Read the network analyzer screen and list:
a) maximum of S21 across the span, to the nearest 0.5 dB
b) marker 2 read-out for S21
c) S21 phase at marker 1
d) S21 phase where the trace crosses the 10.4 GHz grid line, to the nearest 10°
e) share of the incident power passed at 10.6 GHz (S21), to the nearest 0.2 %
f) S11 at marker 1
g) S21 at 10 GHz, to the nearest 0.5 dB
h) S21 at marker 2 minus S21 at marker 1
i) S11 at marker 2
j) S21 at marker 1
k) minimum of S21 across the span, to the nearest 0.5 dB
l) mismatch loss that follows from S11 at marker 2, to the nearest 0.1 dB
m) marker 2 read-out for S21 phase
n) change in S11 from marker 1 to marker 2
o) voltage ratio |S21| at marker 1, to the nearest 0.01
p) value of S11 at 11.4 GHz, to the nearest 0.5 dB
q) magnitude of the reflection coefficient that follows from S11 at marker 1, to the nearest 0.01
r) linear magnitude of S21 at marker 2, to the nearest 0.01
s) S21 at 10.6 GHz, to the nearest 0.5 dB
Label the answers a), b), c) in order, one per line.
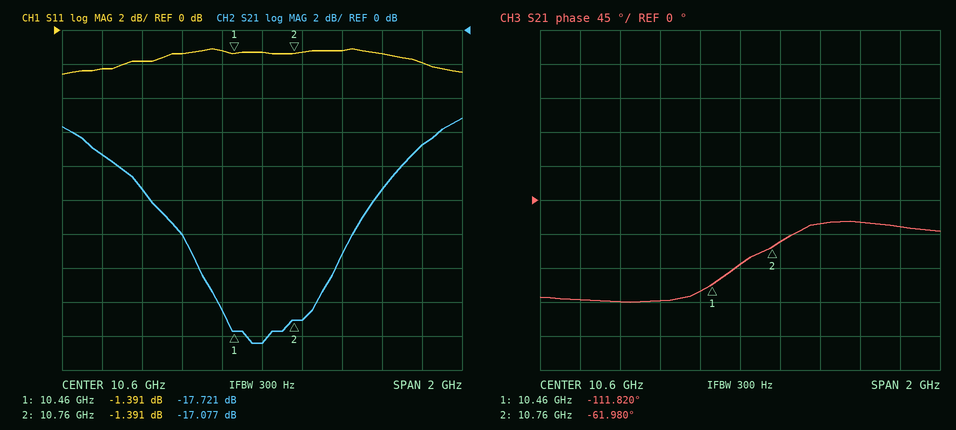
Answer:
a) -5.0 dB
b) -17.077 dB
c) -111.820°
d) -120°
e) 1.4 %
f) -1.391 dB
g) -9.5 dB
h) 0.644 dB
i) -1.391 dB
j) -17.721 dB
k) -18.5 dB
l) 5.6 dB
m) -61.980°
n) 0.000 dB
o) 0.13
p) -2.0 dB
q) 0.85
r) 0.14
s) -18.5 dB
